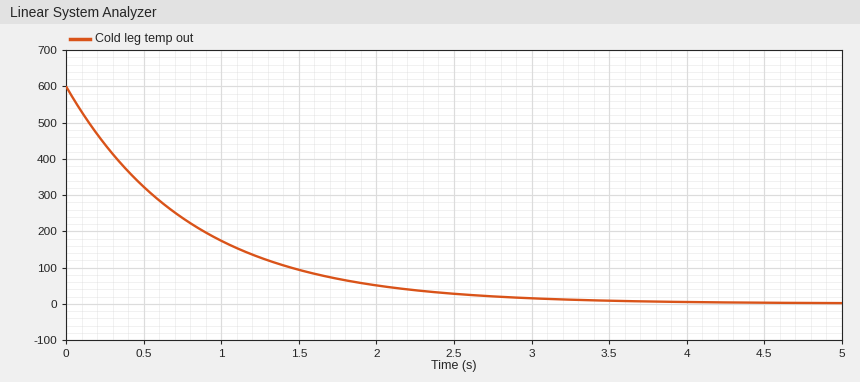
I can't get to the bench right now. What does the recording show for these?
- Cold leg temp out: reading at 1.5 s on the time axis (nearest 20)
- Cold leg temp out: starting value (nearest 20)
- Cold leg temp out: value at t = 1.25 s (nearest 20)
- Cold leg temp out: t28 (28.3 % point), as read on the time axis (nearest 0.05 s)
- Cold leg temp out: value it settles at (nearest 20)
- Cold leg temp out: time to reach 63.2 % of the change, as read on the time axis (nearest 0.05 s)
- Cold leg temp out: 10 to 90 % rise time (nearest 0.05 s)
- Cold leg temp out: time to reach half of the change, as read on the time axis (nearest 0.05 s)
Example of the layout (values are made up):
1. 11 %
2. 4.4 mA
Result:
1. 100
2. 600
3. 120
4. 0.25 s
5. 0
6. 0.80 s
7. 1.75 s
8. 0.55 s
